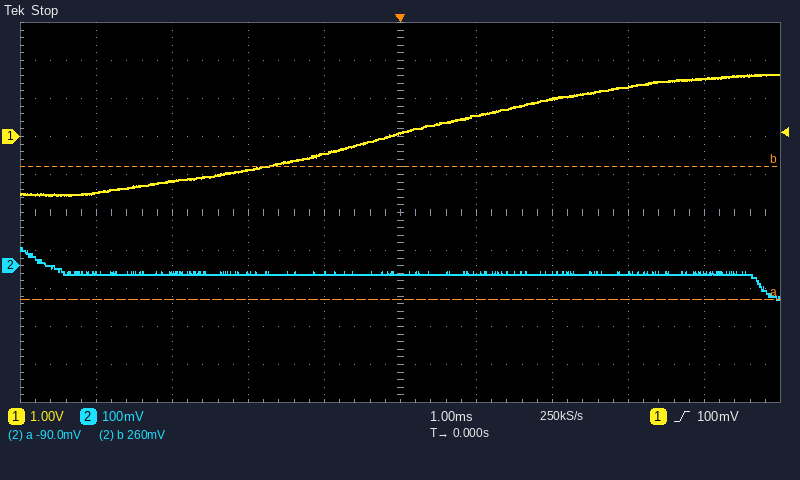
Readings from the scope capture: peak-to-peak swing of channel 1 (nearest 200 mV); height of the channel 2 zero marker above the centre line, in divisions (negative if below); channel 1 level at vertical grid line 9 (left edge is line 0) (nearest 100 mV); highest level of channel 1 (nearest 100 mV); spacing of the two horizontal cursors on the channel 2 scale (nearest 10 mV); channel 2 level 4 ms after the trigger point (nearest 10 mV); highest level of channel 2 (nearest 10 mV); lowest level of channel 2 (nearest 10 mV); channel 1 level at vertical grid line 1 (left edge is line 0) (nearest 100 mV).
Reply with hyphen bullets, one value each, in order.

- 3.2 V
- -1.4 div
- 1.5 V
- 1.6 V
- 350 mV
- -20 mV
- 50 mV
- -90 mV
- -1.5 V
